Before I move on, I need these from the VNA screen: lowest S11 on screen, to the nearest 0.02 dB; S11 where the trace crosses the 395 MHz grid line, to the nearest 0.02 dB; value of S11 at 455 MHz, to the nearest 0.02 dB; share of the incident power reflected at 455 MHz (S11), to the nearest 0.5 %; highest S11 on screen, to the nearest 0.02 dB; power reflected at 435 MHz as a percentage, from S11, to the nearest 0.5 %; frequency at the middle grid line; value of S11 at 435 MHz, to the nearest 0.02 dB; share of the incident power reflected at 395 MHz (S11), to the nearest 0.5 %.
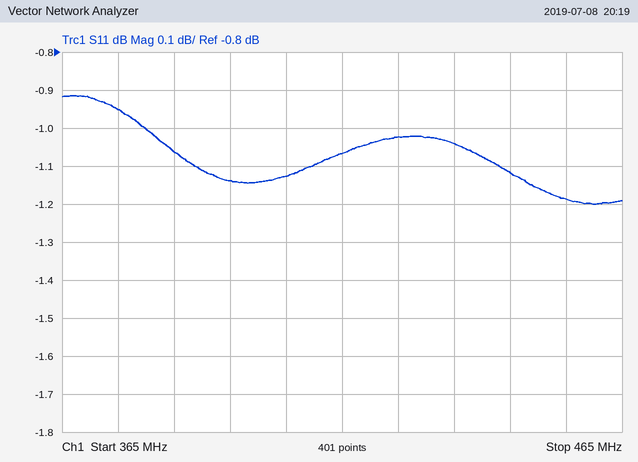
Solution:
-1.20 dB
-1.14 dB
-1.18 dB
76.0 %
-0.92 dB
78.5 %
415 MHz
-1.04 dB
77.0 %
